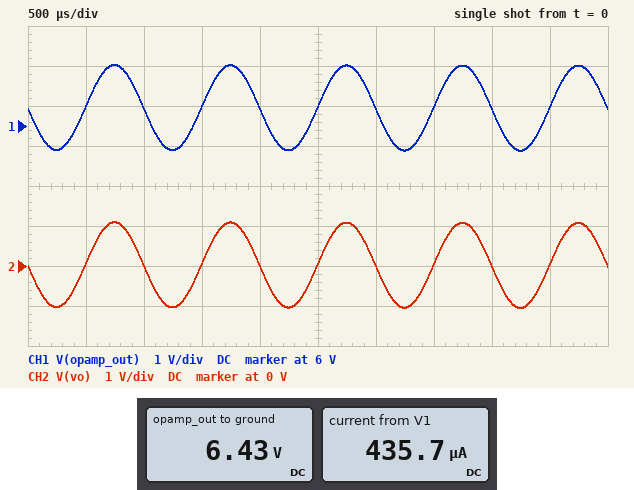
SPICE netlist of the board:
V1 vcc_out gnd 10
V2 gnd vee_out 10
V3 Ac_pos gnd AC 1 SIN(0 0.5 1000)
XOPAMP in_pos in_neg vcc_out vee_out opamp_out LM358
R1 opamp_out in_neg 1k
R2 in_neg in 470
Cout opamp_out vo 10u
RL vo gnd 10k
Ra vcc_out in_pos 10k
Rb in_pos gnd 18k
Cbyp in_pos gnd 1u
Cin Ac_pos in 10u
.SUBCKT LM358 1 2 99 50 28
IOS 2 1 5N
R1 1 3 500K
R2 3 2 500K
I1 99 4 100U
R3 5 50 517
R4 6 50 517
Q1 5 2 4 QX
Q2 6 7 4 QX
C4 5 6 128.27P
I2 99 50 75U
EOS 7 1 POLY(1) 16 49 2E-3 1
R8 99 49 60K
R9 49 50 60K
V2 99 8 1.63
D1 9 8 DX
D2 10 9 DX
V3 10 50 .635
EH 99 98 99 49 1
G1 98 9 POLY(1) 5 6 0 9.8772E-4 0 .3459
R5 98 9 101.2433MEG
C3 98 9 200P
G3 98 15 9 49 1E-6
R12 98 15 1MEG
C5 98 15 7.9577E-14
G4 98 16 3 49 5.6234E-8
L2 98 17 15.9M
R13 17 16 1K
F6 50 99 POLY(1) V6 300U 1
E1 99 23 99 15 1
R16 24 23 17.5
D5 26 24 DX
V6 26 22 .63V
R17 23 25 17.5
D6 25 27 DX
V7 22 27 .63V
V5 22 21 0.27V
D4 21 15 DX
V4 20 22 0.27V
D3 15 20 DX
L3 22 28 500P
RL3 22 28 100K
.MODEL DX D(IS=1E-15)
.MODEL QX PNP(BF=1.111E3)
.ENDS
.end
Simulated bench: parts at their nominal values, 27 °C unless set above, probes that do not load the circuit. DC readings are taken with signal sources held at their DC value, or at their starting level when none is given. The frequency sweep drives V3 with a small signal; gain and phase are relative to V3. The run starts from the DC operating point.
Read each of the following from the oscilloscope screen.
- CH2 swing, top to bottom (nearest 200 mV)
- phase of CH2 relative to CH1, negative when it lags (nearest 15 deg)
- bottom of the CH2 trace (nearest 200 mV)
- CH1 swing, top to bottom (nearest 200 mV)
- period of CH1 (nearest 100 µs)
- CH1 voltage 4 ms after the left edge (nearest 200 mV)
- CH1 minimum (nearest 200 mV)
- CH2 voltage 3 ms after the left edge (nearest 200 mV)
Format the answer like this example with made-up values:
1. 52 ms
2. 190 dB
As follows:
1. 2.2 V
2. 0 deg
3. -1.0 V
4. 2.2 V
5. 1.0 ms
6. 6.4 V
7. 5.4 V
8. 0 V
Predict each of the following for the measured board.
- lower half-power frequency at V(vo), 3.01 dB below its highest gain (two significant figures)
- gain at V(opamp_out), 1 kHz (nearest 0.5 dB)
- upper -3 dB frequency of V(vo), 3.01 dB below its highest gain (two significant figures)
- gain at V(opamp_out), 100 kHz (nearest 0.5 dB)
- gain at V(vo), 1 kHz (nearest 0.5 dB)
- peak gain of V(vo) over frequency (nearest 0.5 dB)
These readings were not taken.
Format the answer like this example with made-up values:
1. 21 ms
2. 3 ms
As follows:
1. 34 Hz
2. 6.5 dB
3. 290 kHz
4. 6.0 dB
5. 6.5 dB
6. 6.5 dB
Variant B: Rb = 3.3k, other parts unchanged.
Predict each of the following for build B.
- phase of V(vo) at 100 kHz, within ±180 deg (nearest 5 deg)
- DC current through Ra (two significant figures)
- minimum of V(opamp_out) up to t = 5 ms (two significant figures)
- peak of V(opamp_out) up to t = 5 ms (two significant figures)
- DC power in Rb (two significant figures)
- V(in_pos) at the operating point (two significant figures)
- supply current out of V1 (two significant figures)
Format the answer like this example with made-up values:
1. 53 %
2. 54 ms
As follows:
1. 150 deg
2. 750 µA
3. 1.4 V
4. 3.6 V
5. 1.9 mW
6. 2.5 V
7. 830 µA
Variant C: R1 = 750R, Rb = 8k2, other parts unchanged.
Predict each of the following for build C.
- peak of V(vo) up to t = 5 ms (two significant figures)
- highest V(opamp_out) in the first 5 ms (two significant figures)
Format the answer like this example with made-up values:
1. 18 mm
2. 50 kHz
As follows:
1. 820 mV
2. 5.3 V
